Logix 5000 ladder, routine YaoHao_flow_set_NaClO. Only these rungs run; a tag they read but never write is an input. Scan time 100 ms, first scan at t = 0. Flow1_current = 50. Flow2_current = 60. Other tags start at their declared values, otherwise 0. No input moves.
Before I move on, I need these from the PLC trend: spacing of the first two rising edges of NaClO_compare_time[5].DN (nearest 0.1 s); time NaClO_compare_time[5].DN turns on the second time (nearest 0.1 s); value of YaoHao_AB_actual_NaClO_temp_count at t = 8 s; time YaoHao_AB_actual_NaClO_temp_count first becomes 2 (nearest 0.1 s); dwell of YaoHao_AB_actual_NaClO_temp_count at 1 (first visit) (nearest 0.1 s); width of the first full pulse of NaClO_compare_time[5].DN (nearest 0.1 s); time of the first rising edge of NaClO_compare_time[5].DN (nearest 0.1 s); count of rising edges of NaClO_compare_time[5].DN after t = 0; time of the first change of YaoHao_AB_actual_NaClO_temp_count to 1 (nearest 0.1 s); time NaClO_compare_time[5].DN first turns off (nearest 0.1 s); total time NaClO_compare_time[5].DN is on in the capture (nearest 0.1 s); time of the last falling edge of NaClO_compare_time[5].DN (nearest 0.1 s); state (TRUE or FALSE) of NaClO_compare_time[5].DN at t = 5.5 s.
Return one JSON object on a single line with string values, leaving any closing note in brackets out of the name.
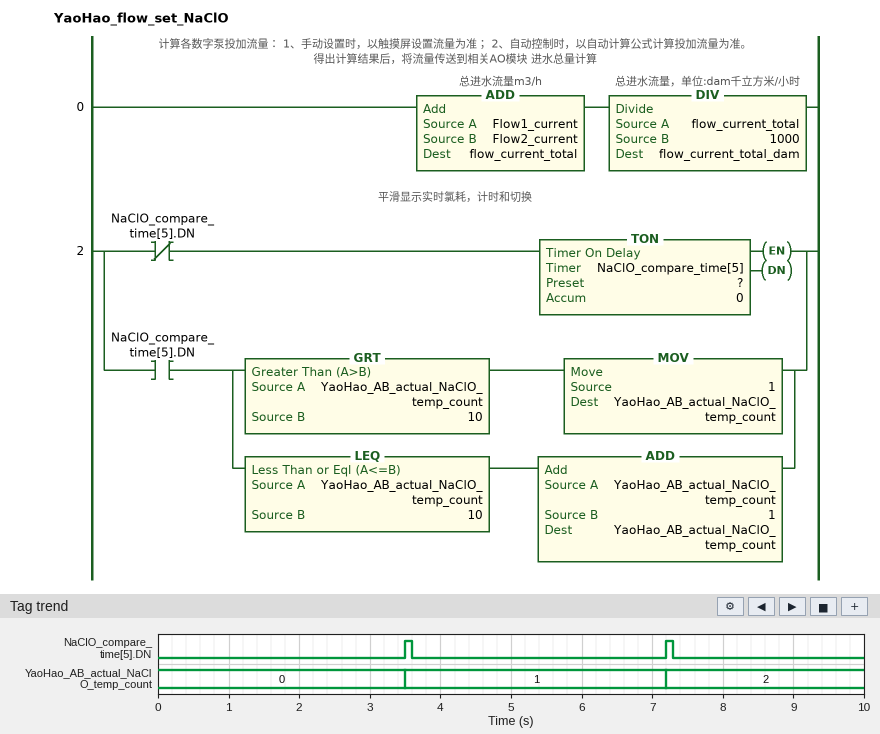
{"spacing of the first two rising edges of NaClO_compare_time[5].DN": "3.7 s", "time NaClO_compare_time[5].DN turns on the second time": "7.2 s", "value of YaoHao_AB_actual_NaClO_temp_count at t = 8 s": "2", "time YaoHao_AB_actual_NaClO_temp_count first becomes 2": "7.2 s", "dwell of YaoHao_AB_actual_NaClO_temp_count at 1 (first visit)": "3.7 s", "width of the first full pulse of NaClO_compare_time[5].DN": "0.1 s", "time of the first rising edge of NaClO_compare_time[5].DN": "3.5 s", "count of rising edges of NaClO_compare_time[5].DN after t = 0": "2", "time of the first change of YaoHao_AB_actual_NaClO_temp_count to 1": "3.5 s", "time NaClO_compare_time[5].DN first turns off": "3.6 s", "total time NaClO_compare_time[5].DN is on in the capture": "0.2 s", "time of the last falling edge of NaClO_compare_time[5].DN": "7.3 s", "state (TRUE or FALSE) of NaClO_compare_time[5].DN at t = 5.5 s": "FALSE"}
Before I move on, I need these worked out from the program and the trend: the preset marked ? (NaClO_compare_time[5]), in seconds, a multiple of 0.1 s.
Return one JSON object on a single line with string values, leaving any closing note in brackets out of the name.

{"the preset marked ? (NaClO_compare_time[5]), in seconds, a multiple of 0.1 s": "3.5 s"}
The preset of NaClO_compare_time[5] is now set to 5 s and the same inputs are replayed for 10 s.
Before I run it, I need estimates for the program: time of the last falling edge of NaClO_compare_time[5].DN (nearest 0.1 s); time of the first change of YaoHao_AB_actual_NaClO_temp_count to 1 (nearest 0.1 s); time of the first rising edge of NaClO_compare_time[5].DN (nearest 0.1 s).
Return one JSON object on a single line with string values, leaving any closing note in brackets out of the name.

{"time of the last falling edge of NaClO_compare_time[5].DN": "5.1 s", "time of the first change of YaoHao_AB_actual_NaClO_temp_count to 1": "5.0 s", "time of the first rising edge of NaClO_compare_time[5].DN": "5.0 s"}
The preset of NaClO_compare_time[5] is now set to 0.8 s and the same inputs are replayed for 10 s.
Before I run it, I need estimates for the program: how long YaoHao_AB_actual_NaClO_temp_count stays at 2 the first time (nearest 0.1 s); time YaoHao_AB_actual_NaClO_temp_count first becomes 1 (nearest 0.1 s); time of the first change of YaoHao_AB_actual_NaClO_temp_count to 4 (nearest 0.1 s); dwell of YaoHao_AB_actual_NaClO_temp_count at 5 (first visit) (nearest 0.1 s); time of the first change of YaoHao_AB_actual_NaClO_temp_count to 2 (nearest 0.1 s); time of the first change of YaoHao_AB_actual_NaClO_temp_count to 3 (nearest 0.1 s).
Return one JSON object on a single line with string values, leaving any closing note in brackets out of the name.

{"how long YaoHao_AB_actual_NaClO_temp_count stays at 2 the first time": "1.0 s", "time YaoHao_AB_actual_NaClO_temp_count first becomes 1": "0.8 s", "time of the first change of YaoHao_AB_actual_NaClO_temp_count to 4": "3.8 s", "dwell of YaoHao_AB_actual_NaClO_temp_count at 5 (first visit)": "1.0 s", "time of the first change of YaoHao_AB_actual_NaClO_temp_count to 2": "1.8 s", "time of the first change of YaoHao_AB_actual_NaClO_temp_count to 3": "2.8 s"}
